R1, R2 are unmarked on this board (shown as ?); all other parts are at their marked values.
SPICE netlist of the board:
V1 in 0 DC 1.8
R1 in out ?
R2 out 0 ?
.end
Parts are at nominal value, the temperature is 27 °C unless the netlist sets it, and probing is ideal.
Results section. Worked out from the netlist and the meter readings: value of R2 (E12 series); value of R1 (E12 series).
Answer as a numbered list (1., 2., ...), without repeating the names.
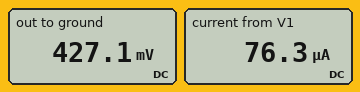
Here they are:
1. 5.6 kΩ
2. 18 kΩ
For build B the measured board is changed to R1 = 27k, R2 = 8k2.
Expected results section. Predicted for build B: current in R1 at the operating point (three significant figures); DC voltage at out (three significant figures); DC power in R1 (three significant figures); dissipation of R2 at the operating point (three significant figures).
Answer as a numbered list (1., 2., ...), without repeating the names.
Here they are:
1. 51.1 µA
2. 419 mV
3. 70.6 µW
4. 21.4 µW
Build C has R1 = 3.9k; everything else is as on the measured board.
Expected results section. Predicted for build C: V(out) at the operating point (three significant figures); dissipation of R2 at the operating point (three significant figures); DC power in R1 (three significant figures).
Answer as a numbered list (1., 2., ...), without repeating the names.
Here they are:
1. 1.06 V
2. 201 µW
3. 140 µW
